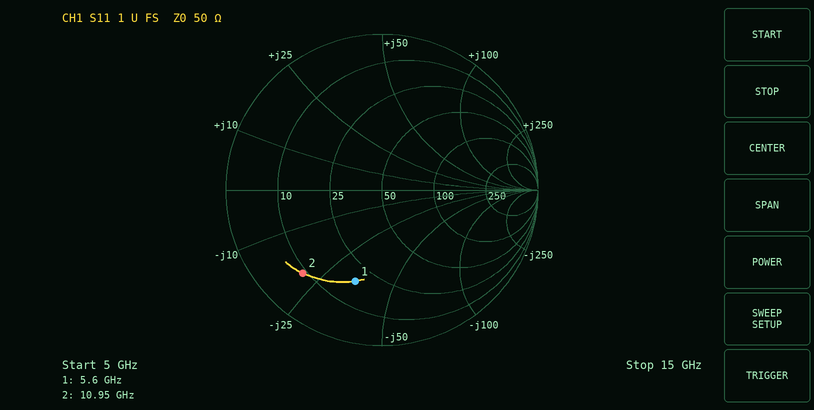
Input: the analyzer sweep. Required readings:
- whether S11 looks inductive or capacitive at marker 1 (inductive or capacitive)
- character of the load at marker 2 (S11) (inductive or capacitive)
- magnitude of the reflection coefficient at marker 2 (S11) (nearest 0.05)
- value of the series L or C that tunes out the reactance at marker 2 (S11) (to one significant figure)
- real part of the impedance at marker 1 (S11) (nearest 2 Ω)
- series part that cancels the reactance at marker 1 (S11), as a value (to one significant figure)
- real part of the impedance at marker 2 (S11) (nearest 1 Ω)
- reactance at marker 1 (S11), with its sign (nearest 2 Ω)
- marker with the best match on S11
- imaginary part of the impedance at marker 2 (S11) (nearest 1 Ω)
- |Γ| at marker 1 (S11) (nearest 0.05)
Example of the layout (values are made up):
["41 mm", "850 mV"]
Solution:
["capacitive", "capacitive", "0.75", "300 pH", "18 Ω", "1.0 nH", "9 Ω", "-34 Ω", "marker 1", "-21 Ω", "0.60"]
